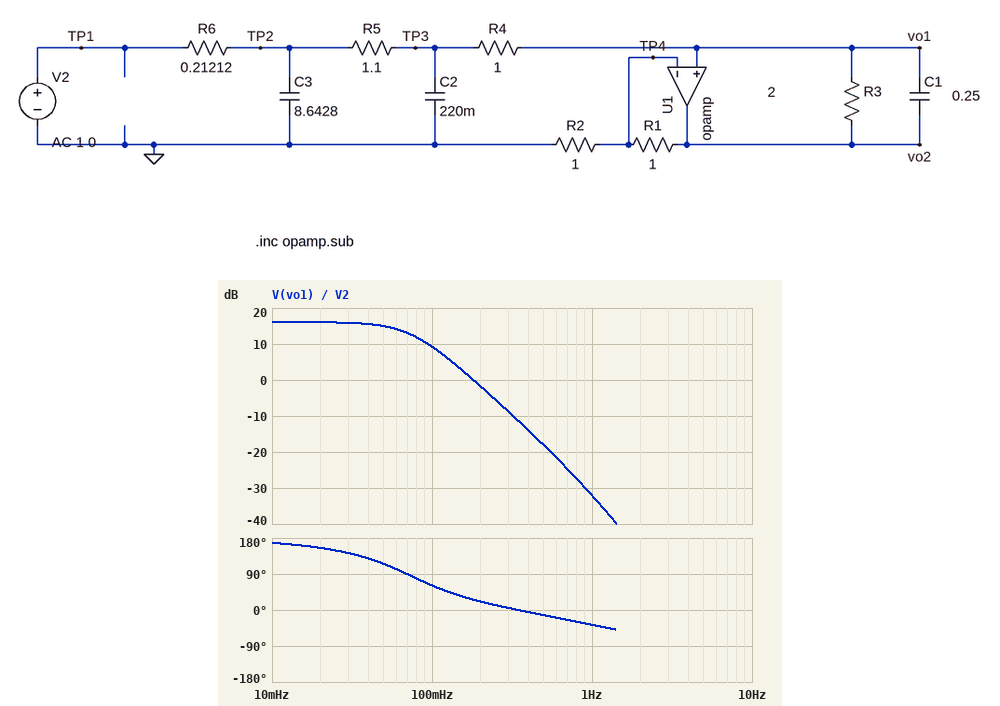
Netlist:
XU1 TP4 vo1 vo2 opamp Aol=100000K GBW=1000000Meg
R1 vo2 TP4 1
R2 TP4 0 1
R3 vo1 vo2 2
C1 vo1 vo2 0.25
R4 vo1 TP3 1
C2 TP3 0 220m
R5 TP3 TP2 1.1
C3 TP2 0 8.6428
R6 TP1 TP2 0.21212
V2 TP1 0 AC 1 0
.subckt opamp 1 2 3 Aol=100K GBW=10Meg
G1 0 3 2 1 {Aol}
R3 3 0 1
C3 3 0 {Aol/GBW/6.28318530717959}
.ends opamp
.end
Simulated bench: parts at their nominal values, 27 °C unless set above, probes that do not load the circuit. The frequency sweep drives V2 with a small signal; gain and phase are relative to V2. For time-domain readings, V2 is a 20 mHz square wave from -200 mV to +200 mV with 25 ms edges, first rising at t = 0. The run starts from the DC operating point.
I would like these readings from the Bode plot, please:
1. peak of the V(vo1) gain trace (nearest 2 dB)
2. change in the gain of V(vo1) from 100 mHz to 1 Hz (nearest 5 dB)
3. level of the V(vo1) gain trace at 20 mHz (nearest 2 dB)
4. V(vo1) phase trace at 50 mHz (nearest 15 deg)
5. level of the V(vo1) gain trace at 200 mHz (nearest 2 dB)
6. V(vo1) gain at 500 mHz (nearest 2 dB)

16 dB
-40 dB
16 dB
120 deg
-2 dB
-18 dB
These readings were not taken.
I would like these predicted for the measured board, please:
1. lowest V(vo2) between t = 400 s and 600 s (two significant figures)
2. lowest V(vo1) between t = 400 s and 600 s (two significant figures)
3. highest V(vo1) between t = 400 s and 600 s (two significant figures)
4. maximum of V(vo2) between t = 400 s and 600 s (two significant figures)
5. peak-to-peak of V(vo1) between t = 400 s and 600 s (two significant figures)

-2.7 V
-1.4 V
1.4 V
2.7 V
2.7 V
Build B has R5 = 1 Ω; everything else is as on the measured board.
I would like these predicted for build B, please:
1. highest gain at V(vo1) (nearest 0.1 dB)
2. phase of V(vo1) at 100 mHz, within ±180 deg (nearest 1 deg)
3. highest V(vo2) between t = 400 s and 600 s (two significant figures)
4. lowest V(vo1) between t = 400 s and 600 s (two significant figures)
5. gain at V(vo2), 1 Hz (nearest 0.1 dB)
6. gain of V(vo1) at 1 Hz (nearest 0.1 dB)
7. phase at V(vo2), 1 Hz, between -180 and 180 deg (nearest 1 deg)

19.5 dB
50 deg
4.0 V
-2.0 V
-25.6 dB
-31.6 dB
-36 deg
